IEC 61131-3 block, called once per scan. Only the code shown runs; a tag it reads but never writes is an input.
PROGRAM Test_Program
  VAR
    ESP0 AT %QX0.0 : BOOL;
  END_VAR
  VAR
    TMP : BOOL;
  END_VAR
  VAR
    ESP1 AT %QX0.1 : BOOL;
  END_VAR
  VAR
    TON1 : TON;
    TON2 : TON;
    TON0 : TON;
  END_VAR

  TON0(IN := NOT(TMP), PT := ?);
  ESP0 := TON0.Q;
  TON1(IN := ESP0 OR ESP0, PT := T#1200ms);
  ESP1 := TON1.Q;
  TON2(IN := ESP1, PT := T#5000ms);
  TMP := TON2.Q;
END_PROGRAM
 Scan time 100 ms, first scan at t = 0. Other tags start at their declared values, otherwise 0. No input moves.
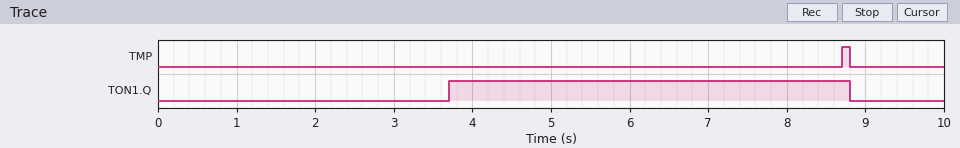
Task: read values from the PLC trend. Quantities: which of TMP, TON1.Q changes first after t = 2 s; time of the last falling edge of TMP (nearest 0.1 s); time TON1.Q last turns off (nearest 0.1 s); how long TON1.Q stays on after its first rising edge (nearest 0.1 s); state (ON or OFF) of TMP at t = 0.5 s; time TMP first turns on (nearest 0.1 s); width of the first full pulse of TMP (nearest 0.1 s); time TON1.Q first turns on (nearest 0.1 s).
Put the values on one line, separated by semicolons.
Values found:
TON1.Q; 8.8 s; 8.8 s; 5.1 s; OFF; 8.7 s; 0.1 s; 3.7 s
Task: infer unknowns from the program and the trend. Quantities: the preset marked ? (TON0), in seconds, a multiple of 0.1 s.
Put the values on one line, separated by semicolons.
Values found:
2.5 s
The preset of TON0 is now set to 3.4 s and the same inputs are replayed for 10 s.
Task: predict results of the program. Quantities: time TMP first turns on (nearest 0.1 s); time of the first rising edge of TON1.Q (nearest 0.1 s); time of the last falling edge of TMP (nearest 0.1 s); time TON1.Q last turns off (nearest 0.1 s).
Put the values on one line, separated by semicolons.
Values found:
9.6 s; 4.6 s; 9.7 s; 9.7 s
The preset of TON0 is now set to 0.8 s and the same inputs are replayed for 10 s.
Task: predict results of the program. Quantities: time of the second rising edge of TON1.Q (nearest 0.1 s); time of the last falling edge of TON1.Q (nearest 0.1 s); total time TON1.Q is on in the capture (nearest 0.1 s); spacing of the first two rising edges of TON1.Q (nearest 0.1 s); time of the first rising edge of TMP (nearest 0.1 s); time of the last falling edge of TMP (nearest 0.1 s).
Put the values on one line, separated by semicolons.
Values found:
9.2 s; 7.1 s; 5.9 s; 7.2 s; 7.0 s; 7.1 s
